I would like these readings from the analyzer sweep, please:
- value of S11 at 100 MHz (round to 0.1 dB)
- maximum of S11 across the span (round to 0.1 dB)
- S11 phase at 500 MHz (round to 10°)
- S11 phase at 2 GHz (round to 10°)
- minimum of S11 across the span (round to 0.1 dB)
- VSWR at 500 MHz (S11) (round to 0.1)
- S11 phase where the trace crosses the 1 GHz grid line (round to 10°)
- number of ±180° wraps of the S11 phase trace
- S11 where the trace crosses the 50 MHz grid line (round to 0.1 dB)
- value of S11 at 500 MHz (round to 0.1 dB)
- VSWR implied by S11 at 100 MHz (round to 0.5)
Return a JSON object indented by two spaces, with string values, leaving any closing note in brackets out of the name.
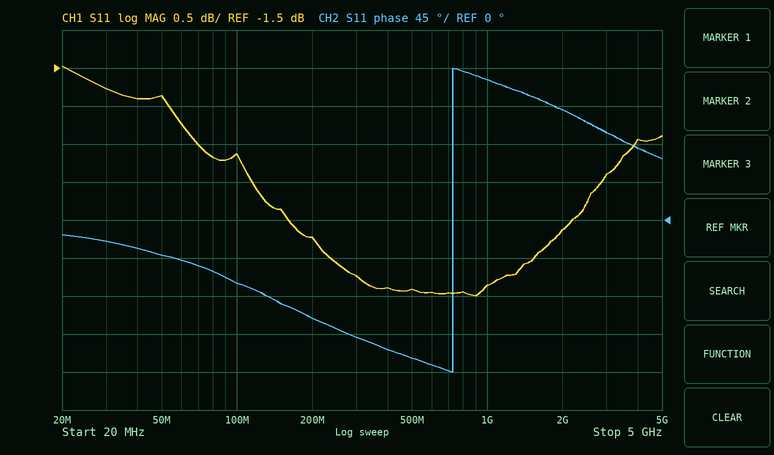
{
  "value of S11 at 100 MHz": "-2.6 dB",
  "maximum of S11 across the span": "-1.5 dB",
  "S11 phase at 500 MHz": "-160°",
  "S11 phase at 2 GHz": "130°",
  "minimum of S11 across the span": "-4.5 dB",
  "VSWR at 500 MHz (S11)": "4.0",
  "S11 phase where the trace crosses the 1 GHz grid line": "170°",
  "number of ±180° wraps of the S11 phase trace": "1",
  "S11 where the trace crosses the 50 MHz grid line": "-1.9 dB",
  "value of S11 at 500 MHz": "-4.4 dB",
  "VSWR implied by S11 at 100 MHz": "6.5"
}
